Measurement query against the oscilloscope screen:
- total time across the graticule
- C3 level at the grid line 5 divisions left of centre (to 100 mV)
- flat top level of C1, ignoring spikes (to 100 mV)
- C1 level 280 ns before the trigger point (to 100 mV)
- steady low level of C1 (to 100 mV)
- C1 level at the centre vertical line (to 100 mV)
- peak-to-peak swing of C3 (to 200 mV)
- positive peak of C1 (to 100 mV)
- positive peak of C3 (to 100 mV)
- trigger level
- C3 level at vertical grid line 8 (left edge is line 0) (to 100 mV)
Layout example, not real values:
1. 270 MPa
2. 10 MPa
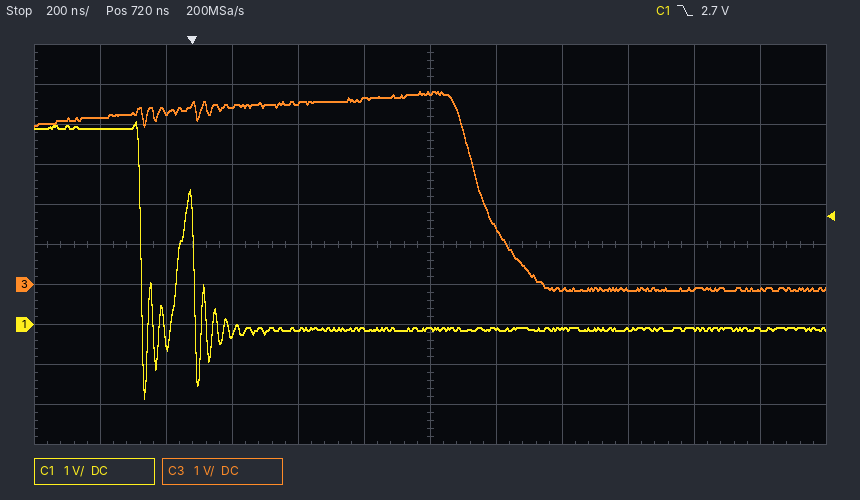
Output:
1. 2.4 µs
2. 4.2 V
3. 4.9 V
4. 4.9 V
5. -100 mV
6. -100 mV
7. 5.0 V
8. 5.1 V
9. 4.8 V
10. 2.7 V
11. -100 mV
